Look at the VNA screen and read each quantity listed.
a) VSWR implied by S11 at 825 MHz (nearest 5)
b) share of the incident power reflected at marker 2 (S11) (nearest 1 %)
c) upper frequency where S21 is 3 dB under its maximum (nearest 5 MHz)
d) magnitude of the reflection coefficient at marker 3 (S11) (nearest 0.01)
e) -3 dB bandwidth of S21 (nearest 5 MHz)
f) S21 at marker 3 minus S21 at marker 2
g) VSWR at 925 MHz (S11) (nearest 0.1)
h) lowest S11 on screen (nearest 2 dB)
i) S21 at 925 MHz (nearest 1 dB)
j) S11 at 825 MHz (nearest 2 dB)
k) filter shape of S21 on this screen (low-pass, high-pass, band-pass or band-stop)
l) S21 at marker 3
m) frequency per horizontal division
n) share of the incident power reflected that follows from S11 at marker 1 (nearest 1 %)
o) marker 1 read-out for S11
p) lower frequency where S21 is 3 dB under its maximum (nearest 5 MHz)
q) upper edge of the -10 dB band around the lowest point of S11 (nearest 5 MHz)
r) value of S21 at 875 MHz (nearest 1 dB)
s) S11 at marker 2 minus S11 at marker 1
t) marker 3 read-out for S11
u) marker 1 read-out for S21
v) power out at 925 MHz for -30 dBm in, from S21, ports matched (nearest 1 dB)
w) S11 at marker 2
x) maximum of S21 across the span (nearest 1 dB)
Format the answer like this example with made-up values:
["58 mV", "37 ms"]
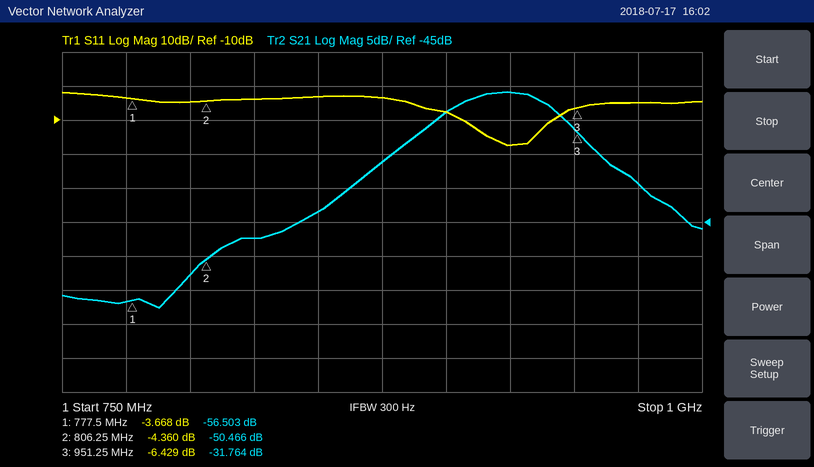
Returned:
["5", "37 %", "945 MHz", "0.48", "45 MHz", "18.702 dB", "1.3", "-18 dB", "-26 dB", "-4 dB", "band-pass", "-31.764 dB", "25 MHz", "43 %", "-3.668 dB", "900 MHz", "940 MHz", "-36 dB", "-0.692 dB", "-6.429 dB", "-56.503 dB", "-56 dBm", "-4.360 dB", "-26 dB"]
